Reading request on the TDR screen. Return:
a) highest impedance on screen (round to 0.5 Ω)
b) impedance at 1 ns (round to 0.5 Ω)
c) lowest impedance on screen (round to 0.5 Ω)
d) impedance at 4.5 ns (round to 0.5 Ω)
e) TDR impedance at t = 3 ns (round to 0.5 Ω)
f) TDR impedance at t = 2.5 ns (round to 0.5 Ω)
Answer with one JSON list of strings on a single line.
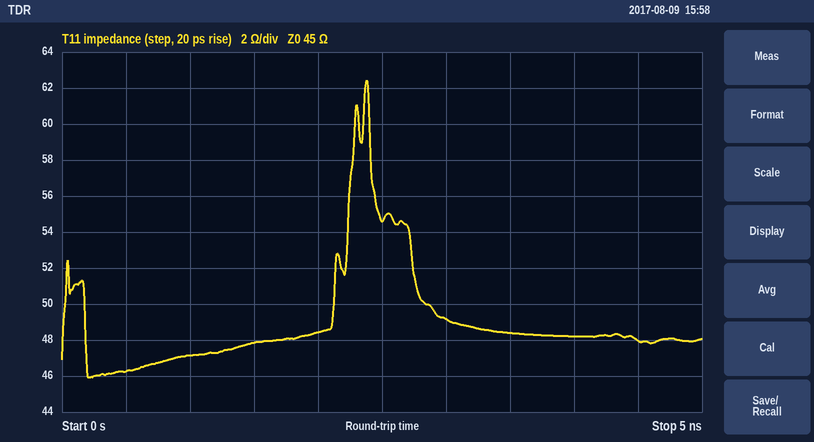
["62.5 Ω", "47.0 Ω", "46.0 Ω", "48.0 Ω", "49.0 Ω", "54.5 Ω"]
